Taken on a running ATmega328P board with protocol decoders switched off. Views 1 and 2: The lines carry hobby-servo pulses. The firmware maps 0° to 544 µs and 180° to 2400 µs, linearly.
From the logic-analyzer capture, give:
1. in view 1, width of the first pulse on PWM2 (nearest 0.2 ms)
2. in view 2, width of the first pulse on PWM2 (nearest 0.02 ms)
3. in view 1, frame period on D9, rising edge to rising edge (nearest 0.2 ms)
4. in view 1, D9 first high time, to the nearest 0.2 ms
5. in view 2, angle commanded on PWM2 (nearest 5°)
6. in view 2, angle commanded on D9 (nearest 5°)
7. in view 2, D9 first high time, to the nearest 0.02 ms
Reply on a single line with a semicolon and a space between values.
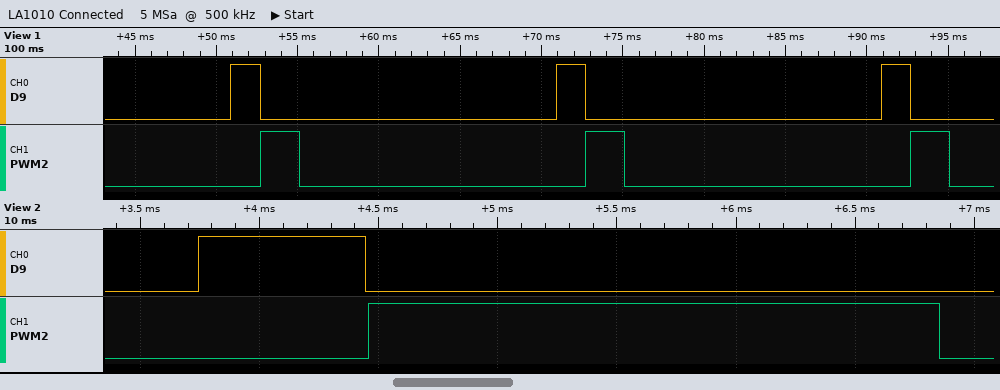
2.4 ms; 2.40 ms; 20.0 ms; 1.8 ms; 180°; 15°; 0.70 ms
